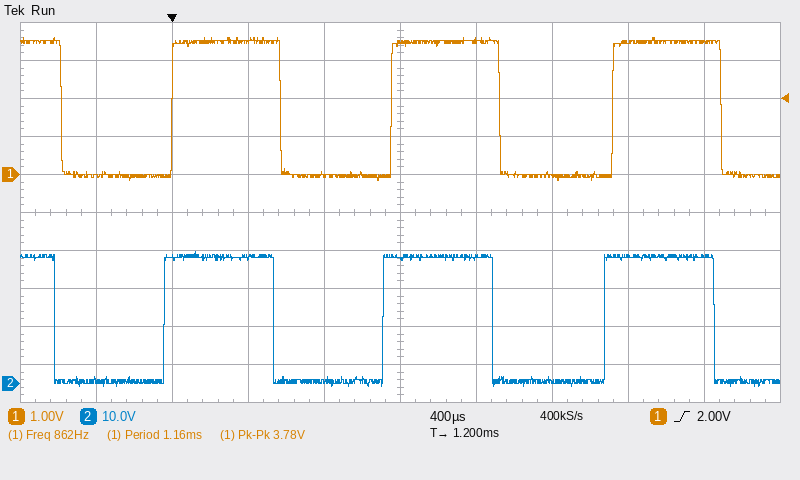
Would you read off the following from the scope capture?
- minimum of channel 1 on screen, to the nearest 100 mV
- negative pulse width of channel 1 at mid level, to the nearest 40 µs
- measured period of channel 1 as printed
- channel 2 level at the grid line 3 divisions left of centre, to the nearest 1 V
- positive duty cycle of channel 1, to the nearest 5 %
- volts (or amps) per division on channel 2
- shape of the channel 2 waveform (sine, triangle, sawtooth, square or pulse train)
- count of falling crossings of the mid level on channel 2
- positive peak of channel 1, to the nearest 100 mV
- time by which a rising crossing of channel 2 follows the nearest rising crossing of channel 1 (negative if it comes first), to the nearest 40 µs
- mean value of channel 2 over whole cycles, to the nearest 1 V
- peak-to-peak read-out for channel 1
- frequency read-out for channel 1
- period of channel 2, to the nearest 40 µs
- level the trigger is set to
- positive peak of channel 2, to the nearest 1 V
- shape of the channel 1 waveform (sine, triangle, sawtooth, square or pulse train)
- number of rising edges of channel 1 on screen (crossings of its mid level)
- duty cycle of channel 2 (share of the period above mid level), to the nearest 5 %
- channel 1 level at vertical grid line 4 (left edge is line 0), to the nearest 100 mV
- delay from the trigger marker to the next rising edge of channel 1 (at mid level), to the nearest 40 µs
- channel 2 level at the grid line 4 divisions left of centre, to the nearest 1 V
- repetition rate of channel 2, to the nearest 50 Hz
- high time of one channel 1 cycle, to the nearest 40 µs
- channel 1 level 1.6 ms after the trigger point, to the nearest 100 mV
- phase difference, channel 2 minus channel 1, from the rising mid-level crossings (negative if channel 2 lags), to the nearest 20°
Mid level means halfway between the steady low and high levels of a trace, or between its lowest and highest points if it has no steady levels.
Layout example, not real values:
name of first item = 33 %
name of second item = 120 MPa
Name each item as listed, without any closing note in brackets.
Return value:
minimum of channel 1 on screen, to the nearest 100 mV = -200 mV
negative pulse width of channel 1 at mid level, to the nearest 40 µs = 600 µs
measured period of channel 1 as printed = 1.16 ms
channel 2 level at the grid line 3 divisions left of centre, to the nearest 1 V = 33 V
positive duty cycle of channel 1, to the nearest 5 % = 50 %
volts (or amps) per division on channel 2 = 10 V
shape of the channel 2 waveform = square
count of falling crossings of the mid level on channel 2 = 4
positive peak of channel 1, to the nearest 100 mV = 3.6 V
time by which a rising crossing of channel 2 follows the nearest rising crossing of channel 1 (negative if it comes first), to the nearest 40 µs = -40 µs
mean value of channel 2 over whole cycles, to the nearest 1 V = 17 V
peak-to-peak read-out for channel 1 = 3.78 V
frequency read-out for channel 1 = 862 Hz
period of channel 2, to the nearest 40 µs = 1.16 ms
level the trigger is set to = 2.00 V
positive peak of channel 2, to the nearest 1 V = 35 V
shape of the channel 1 waveform = square
number of rising edges of channel 1 on screen = 3
duty cycle of channel 2 (share of the period above mid level), to the nearest 5 % = 50 %
channel 1 level at vertical grid line 4 (left edge is line 0), to the nearest 100 mV = 0.0 V
delay from the trigger marker to the next rising edge of channel 1 (at mid level), to the nearest 40 µs = 1.16 ms
channel 2 level at the grid line 4 divisions left of centre, to the nearest 1 V = 1 V
repetition rate of channel 2, to the nearest 50 Hz = 850 Hz
high time of one channel 1 cycle, to the nearest 40 µs = 560 µs
channel 1 level 1.6 ms after the trigger point, to the nearest 100 mV = 3.5 V
phase difference, channel 2 minus channel 1, from the rising mid-level crossings (negative if channel 2 lags), to the nearest 20° = +20°
